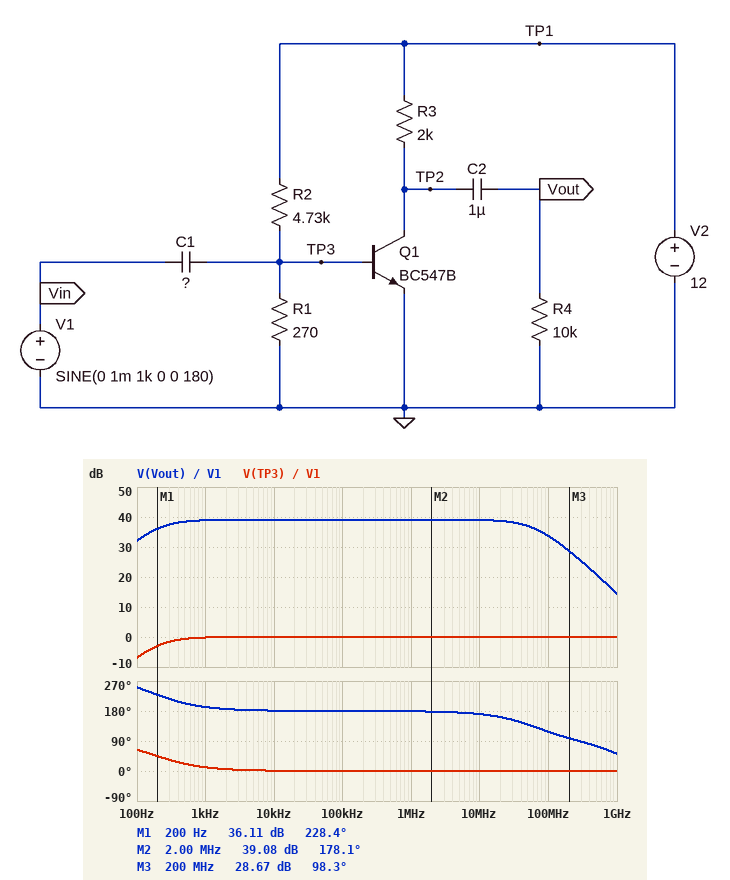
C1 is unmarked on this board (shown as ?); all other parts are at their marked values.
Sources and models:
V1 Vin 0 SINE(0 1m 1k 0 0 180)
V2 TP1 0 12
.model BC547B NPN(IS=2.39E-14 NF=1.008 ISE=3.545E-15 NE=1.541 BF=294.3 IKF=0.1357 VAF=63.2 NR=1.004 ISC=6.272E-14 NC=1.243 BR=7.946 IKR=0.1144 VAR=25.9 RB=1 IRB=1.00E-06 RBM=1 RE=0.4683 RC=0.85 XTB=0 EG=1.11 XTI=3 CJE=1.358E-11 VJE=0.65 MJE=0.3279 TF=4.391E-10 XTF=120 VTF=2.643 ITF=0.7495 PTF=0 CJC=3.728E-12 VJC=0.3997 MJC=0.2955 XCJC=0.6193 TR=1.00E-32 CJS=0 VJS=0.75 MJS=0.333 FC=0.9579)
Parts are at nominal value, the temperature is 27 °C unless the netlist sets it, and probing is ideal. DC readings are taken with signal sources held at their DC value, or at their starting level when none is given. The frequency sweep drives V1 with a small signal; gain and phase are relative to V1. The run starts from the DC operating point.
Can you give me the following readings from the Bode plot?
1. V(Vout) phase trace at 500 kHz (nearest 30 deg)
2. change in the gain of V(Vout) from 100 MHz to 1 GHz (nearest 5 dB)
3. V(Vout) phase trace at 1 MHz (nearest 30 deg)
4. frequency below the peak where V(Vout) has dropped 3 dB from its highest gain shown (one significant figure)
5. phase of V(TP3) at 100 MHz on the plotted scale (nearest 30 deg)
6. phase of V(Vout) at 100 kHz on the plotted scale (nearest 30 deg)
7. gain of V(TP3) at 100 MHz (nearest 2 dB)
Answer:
180 deg
-20 dB
180 deg
200 Hz
0 deg
180 deg
0 dB
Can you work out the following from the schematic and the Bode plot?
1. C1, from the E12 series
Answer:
3.3 µF
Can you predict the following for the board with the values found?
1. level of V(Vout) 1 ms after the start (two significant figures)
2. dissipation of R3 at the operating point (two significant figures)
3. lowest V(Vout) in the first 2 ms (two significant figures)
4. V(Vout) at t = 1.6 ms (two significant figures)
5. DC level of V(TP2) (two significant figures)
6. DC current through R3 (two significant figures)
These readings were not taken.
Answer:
13 mV
4.6 mW
-97 mV
-69 mV
9.0 V
1.5 mA
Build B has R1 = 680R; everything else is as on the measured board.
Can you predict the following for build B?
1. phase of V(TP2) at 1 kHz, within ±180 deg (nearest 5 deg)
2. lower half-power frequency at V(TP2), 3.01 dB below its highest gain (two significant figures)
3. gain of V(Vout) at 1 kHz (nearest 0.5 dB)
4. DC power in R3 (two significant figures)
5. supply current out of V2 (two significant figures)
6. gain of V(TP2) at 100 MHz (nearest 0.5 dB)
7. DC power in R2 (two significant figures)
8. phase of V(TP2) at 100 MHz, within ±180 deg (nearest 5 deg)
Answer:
-105 deg
43 MHz
-17.5 dB
72 mW
8.4 mA
-6.0 dB
27 mW
130 deg
